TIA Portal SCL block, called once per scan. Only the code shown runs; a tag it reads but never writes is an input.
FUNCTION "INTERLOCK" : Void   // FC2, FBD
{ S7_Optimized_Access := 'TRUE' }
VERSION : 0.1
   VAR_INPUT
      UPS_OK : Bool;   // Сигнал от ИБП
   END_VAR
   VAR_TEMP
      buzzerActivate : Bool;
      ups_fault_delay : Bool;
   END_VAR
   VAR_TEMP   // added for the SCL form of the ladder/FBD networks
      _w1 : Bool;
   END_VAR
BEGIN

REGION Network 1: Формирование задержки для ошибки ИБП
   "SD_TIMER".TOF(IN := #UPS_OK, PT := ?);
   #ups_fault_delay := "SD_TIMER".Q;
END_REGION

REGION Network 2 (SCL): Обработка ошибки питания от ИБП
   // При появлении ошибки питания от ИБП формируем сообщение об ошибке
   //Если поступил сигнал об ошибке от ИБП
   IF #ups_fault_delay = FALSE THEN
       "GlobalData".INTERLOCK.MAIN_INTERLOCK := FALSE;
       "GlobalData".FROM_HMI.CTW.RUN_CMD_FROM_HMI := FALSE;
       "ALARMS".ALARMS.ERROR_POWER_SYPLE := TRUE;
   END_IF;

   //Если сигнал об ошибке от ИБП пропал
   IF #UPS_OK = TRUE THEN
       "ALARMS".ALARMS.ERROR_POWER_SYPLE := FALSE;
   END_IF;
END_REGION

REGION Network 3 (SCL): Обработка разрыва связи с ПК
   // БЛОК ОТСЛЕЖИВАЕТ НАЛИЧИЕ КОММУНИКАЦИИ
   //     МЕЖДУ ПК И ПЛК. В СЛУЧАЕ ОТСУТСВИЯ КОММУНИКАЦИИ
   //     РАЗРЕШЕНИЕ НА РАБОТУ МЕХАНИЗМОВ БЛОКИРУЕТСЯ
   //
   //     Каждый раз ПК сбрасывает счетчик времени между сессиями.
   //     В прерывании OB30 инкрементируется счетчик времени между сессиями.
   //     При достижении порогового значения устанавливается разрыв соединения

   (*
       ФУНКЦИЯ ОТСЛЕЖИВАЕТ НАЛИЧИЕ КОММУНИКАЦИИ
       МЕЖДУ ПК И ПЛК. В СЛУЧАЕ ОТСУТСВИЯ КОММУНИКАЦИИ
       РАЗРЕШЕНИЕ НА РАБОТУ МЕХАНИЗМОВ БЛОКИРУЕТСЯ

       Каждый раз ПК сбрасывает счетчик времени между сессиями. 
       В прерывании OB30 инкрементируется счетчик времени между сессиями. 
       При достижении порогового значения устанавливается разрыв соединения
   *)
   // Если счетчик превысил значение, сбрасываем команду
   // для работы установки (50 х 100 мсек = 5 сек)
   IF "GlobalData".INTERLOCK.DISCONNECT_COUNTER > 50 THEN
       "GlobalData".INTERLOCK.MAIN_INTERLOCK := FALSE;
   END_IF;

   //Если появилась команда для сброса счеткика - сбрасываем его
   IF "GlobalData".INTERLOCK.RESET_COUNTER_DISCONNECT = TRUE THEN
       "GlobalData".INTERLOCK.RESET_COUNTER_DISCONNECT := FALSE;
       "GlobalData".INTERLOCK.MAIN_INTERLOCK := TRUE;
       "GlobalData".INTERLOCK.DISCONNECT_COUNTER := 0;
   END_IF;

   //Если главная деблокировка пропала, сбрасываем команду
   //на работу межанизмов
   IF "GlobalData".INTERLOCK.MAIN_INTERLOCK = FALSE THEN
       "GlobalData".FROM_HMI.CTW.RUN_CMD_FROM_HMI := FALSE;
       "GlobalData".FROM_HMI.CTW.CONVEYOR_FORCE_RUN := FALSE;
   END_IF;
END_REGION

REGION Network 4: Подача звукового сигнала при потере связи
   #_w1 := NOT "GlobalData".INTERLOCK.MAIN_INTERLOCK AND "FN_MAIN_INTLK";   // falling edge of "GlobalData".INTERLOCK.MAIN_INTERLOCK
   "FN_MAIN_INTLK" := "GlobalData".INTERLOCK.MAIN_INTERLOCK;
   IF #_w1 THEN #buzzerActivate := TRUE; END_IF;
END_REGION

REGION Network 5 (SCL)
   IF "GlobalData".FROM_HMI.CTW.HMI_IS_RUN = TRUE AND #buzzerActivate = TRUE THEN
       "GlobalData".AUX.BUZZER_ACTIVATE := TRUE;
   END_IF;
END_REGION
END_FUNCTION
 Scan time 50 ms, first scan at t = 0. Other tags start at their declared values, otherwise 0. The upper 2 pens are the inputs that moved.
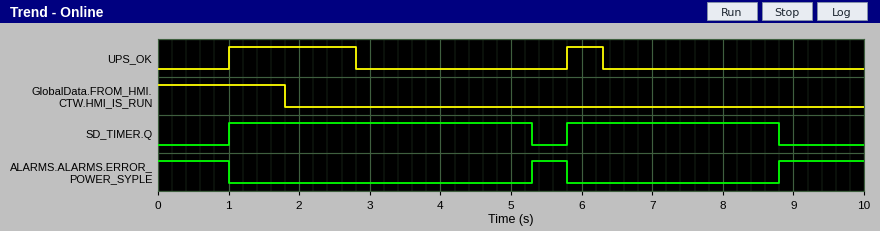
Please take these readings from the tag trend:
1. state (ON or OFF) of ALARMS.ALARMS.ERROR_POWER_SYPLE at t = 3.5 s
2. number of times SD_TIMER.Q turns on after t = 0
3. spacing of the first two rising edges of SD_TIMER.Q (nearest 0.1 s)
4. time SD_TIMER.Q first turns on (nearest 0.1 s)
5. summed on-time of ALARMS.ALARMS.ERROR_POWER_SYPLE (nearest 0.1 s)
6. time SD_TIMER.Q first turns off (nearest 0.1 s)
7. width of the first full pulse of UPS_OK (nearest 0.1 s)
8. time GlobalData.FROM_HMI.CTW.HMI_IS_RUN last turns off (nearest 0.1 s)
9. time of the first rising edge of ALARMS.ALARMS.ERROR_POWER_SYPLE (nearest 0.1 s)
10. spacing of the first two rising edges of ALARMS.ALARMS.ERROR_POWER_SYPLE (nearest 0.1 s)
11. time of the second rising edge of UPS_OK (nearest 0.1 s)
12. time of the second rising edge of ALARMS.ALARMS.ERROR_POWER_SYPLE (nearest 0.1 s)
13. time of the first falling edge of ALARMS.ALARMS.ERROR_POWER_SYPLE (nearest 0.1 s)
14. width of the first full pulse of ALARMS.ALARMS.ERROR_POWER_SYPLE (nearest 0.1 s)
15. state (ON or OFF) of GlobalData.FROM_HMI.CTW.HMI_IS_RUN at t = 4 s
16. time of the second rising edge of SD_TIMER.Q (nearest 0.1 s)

OFF
2
4.8 s
1.0 s
2.7 s
5.3 s
1.8 s
1.8 s
5.3 s
3.5 s
5.8 s
8.8 s
1.0 s
0.5 s
OFF
5.8 s
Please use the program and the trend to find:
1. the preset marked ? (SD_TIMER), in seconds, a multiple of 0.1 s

2.5 s
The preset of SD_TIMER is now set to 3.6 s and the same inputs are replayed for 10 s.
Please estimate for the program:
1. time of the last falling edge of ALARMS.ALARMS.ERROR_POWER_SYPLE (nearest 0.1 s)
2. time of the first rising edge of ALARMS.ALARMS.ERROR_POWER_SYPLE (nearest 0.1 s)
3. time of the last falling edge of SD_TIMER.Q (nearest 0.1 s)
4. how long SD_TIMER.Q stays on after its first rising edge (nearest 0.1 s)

1.0 s
9.9 s
9.9 s
8.9 s
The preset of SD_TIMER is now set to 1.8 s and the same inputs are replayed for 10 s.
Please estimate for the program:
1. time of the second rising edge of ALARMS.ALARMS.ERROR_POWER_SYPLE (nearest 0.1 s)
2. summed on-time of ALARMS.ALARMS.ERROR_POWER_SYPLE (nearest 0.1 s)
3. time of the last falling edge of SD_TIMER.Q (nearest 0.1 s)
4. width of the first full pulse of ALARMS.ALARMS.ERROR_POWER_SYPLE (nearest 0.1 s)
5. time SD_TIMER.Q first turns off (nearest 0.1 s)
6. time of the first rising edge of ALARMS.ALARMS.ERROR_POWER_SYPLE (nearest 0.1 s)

8.1 s
4.1 s
8.1 s
1.2 s
4.6 s
4.6 s
